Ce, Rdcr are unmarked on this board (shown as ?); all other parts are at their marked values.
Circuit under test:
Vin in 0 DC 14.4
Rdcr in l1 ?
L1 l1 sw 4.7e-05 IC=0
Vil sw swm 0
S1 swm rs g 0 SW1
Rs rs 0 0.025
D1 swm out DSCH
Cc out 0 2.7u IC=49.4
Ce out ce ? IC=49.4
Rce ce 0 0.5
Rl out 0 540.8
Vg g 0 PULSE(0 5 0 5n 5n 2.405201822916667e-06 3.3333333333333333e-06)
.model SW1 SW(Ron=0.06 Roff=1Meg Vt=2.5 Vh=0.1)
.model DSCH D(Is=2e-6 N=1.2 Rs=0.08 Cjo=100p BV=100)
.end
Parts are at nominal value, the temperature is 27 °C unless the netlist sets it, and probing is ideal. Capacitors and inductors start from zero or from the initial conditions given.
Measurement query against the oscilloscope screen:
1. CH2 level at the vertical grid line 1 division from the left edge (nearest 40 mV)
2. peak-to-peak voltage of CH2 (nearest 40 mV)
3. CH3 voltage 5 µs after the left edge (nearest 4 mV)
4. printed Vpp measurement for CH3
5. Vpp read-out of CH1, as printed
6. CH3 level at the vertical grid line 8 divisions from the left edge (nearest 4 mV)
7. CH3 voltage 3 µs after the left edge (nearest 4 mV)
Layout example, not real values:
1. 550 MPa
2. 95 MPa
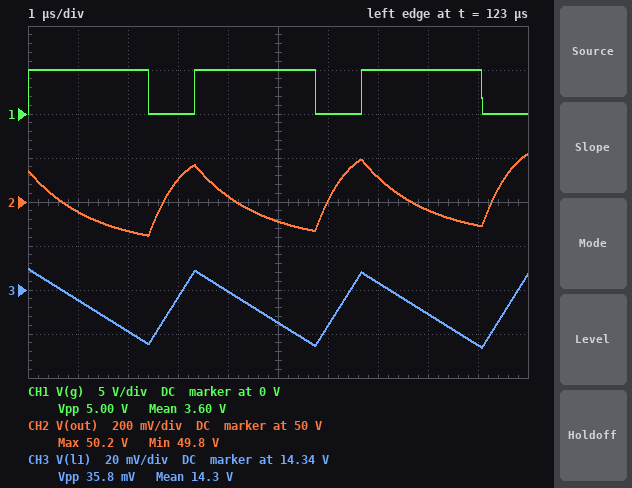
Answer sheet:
1. 49.96 V
2. 360 mV
3. 14.324 V
4. 35.8 mV
5. 5.00 V
6. 14.328 V
7. 14.336 V
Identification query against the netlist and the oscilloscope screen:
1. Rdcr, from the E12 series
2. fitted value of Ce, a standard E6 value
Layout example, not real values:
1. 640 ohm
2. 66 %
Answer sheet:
1. 0.047 Ω
2. 47 µF
